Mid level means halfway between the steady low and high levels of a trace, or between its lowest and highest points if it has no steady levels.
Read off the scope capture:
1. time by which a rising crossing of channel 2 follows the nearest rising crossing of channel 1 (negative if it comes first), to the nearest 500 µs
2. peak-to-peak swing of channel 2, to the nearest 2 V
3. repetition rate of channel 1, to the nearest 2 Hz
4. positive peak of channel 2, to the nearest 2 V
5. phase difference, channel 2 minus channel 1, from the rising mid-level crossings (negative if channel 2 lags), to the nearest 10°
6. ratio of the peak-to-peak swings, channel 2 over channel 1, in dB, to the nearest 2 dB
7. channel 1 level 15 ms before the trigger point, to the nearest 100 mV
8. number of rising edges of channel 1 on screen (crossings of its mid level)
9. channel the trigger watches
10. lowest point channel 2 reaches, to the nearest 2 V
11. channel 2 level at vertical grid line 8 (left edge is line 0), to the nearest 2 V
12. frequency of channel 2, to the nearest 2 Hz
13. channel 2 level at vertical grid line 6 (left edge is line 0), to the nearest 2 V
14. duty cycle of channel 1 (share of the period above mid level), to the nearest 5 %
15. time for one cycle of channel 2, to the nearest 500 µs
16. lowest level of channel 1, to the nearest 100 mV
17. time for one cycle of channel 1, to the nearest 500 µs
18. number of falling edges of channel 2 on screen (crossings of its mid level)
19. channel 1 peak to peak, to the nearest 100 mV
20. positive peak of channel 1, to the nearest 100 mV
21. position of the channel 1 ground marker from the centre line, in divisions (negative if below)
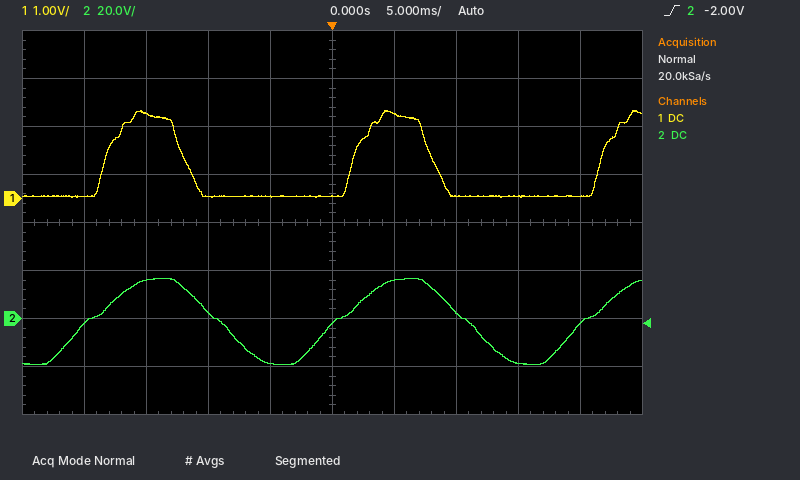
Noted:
-1.5 ms
36 V
50 Hz
16 V
+30°
26 dB
1.8 V
3
channel 2
-20 V
-18 V
50 Hz
16 V
30 %
20.0 ms
0.0 V
20.0 ms
2
1.8 V
1.8 V
+0.5 div
